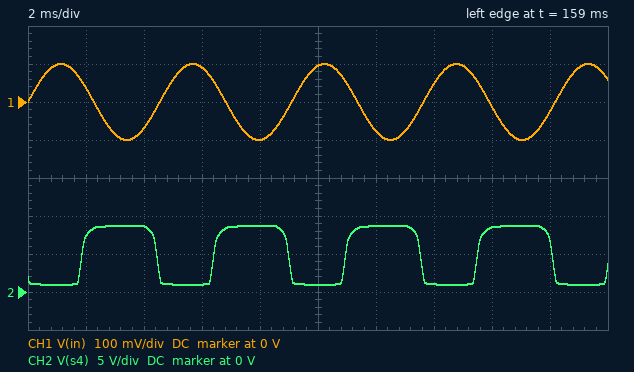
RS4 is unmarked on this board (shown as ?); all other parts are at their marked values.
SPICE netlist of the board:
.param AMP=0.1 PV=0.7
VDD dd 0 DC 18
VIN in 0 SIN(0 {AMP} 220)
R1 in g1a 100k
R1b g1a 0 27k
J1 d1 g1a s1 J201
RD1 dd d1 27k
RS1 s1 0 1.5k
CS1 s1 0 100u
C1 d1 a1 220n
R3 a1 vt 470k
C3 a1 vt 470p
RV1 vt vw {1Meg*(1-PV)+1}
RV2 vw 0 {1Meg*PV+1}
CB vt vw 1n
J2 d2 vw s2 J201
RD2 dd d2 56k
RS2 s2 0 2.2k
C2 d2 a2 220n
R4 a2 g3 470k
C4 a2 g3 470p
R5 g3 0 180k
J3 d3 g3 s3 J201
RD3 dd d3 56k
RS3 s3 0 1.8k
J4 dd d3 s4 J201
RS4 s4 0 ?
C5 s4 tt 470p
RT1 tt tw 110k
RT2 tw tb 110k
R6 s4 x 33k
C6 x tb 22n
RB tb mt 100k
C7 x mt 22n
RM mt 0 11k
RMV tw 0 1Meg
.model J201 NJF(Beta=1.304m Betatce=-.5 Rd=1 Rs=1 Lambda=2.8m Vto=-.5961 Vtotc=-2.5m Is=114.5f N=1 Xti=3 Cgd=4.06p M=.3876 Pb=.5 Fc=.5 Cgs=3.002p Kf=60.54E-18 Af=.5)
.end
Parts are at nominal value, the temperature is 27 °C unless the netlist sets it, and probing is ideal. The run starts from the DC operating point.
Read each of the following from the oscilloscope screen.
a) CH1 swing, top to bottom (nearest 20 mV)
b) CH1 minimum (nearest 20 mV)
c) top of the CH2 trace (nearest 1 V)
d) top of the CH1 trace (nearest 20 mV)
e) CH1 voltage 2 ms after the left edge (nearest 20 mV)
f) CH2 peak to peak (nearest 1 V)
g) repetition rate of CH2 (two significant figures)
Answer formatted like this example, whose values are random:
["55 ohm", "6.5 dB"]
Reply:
["200 mV", "-100 mV", "9 V", "100 mV", "40 mV", "8 V", "220 Hz"]
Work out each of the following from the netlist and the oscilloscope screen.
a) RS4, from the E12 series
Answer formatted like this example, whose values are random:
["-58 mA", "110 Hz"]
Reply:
["4.7 kΩ"]
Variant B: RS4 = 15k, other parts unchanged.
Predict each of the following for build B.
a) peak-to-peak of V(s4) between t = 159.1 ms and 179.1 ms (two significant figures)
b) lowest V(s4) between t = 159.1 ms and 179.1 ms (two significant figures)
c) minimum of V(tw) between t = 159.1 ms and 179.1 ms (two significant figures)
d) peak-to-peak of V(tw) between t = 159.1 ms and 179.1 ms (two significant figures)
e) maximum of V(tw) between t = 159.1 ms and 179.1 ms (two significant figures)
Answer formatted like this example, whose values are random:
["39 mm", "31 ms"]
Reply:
["16 V", "1.3 V", "-4.5 V", "8.9 V", "4.4 V"]
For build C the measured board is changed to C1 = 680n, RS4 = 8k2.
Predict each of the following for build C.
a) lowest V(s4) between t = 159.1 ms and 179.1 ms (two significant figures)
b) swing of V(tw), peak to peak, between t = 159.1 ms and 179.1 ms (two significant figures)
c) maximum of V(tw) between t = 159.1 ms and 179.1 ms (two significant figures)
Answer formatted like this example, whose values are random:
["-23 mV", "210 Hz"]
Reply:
["1.1 V", "7.0 V", "3.3 V"]
